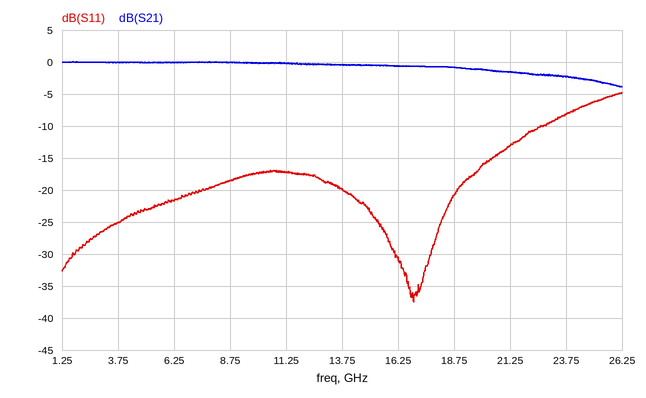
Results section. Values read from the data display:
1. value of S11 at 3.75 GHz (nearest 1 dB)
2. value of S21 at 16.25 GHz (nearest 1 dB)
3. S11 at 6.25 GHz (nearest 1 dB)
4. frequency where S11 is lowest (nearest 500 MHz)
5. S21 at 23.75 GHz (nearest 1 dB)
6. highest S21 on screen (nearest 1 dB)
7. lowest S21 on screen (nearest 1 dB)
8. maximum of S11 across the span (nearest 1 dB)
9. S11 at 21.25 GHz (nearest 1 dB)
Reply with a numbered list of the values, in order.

1. -25 dB
2. -1 dB
3. -22 dB
4. 17.0 GHz
5. -2 dB
6. 0 dB
7. -4 dB
8. -5 dB
9. -13 dB
